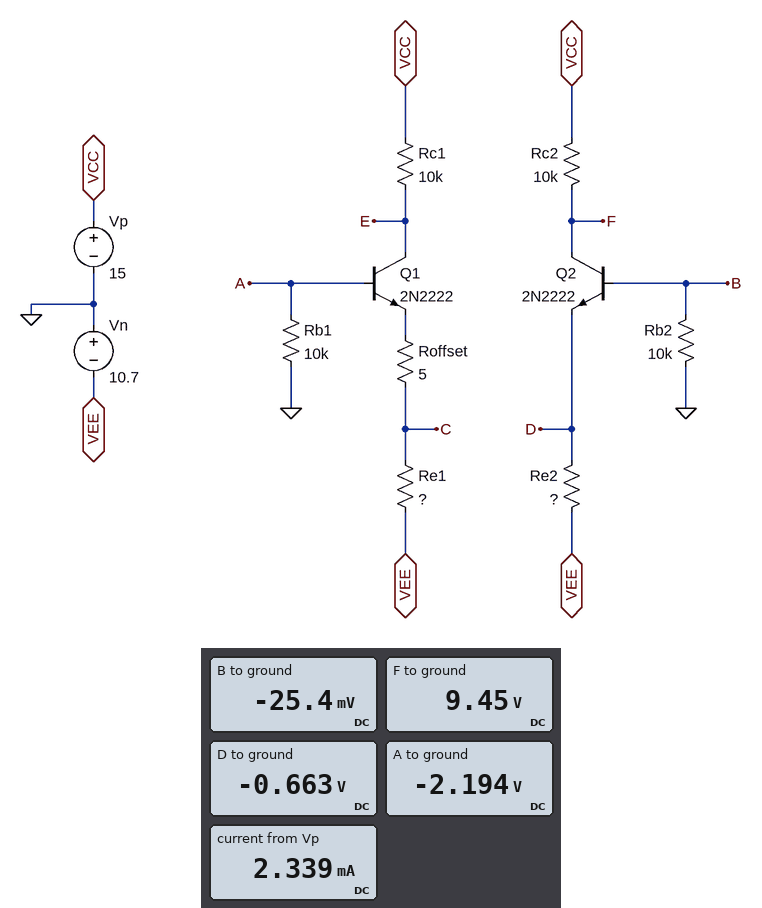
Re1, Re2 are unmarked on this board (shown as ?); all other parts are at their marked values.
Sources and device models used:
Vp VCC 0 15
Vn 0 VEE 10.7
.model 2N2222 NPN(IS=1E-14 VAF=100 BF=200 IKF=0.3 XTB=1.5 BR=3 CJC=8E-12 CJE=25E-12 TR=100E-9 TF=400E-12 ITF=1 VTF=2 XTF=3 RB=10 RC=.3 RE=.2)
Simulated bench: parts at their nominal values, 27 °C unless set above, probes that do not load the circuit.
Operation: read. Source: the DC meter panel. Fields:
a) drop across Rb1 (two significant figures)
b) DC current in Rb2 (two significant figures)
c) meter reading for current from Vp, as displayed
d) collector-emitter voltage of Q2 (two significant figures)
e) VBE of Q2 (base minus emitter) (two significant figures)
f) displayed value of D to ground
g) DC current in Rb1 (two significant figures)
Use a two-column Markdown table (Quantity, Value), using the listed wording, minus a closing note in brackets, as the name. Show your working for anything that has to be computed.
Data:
| Quantity | Value |
|---|---|
| drop across Rb1 | 0 V - (-2.194 V) = 2.2 V |
| DC current in Rb2 | (0 V - (-25.4 mV)) / 10 kΩ = 2.5 µA |
| meter reading for current from Vp, as displayed | 2.339 mA |
| collector-emitter voltage of Q2 | 9.45 V - (-663 mV) = 10 V |
| VBE of Q2 (base minus emitter) | -25.4 mV - (-663 mV) = 640 mV |
| displayed value of D to ground | -0.663 V |
| DC current in Rb1 | (0 V - (-2.194 V)) / 10 kΩ = 220 µA |
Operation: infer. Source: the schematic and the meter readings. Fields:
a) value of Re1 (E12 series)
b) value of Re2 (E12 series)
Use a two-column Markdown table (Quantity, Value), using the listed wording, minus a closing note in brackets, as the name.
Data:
| Quantity | Value |
|---|---|
| value of Re1 | 3.9 kΩ |
| value of Re2 | 18 kΩ |
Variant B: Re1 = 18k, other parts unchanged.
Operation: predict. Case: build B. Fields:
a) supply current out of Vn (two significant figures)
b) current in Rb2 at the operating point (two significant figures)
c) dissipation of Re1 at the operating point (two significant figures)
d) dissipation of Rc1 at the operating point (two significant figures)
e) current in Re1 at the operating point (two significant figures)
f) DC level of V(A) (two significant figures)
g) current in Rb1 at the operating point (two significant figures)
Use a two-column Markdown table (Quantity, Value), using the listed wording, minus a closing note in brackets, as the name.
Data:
| Quantity | Value |
|---|---|
| supply current out of Vn | 1.1 mA |
| current in Rb2 at the operating point | 2.5 µA |
| dissipation of Re1 at the operating point | 5.6 mW |
| dissipation of Rc1 at the operating point | 3.1 mW |
| current in Re1 at the operating point | 560 µA |
| DC level of V(A) | -25 mV |
| current in Rb1 at the operating point | 2.5 µA |
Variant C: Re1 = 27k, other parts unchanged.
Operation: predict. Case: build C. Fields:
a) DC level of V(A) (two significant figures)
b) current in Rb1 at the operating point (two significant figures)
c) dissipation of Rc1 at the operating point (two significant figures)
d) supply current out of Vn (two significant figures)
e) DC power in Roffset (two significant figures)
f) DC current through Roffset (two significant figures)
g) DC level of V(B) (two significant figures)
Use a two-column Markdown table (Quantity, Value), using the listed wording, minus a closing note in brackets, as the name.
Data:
| Quantity | Value |
|---|---|
| DC level of V(A) | -17 mV |
| current in Rb1 at the operating point | 1.7 µA |
| dissipation of Rc1 at the operating point | 1.4 mW |
| supply current out of Vn | 930 µA |
| DC power in Roffset | 690 nW |
| DC current through Roffset | 370 µA |
| DC level of V(B) | -25 mV |
